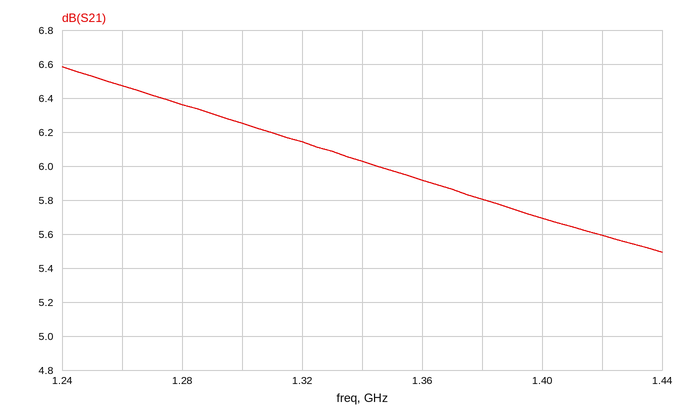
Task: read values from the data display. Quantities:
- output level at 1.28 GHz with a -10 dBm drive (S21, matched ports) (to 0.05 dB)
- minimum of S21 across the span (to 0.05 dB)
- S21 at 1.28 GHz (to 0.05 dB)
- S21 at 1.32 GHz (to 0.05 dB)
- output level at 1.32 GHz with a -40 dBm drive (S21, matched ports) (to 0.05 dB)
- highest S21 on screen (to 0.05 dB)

-3.65 dBm
5.50 dB
6.35 dB
6.15 dB
-33.85 dBm
6.60 dB
